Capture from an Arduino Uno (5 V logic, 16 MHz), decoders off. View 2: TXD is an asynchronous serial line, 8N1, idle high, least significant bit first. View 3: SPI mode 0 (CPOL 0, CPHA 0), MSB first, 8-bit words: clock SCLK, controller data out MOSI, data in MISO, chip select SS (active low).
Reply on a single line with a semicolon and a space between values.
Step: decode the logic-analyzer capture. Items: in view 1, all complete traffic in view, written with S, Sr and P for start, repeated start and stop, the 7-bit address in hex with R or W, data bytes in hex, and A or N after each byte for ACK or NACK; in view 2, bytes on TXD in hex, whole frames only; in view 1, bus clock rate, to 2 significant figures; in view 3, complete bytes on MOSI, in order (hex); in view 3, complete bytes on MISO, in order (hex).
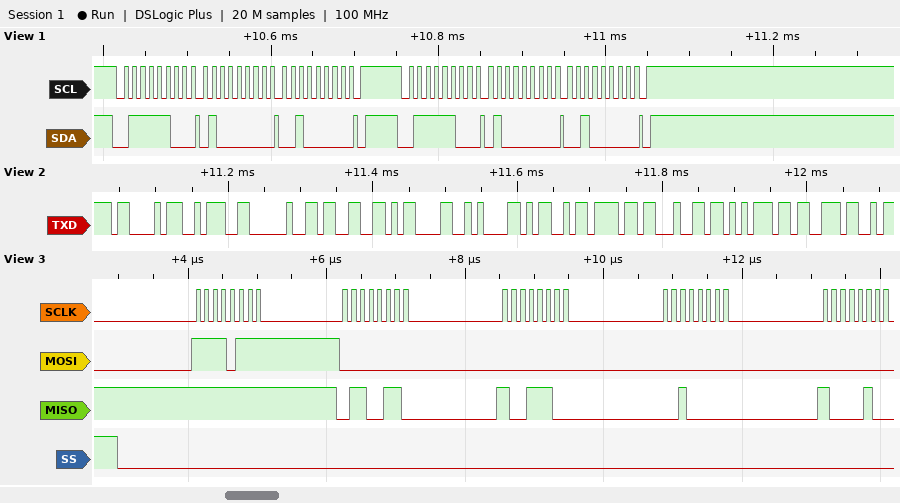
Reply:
S 3EW A 40 A 20 A P S 3EW A 40 A 20 A P; 0x43 0x3A 0x20 0x33 0x0D 0x0A 0x4D 0x6F 0x64 0x75 0x73; 100 kHz; F7 00 00 00 00; FF 66 9C 20 84
